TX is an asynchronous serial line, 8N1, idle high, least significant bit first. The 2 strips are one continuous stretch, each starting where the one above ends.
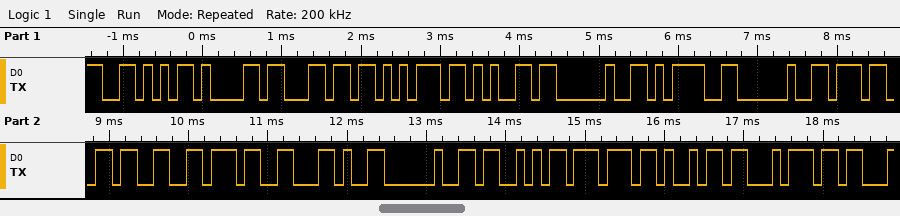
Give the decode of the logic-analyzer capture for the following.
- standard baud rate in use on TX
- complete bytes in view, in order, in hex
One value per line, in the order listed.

9600 baud
56 61 6C 75 65 20 3D 20 37 33 37 2C 20 53 77 69 74
